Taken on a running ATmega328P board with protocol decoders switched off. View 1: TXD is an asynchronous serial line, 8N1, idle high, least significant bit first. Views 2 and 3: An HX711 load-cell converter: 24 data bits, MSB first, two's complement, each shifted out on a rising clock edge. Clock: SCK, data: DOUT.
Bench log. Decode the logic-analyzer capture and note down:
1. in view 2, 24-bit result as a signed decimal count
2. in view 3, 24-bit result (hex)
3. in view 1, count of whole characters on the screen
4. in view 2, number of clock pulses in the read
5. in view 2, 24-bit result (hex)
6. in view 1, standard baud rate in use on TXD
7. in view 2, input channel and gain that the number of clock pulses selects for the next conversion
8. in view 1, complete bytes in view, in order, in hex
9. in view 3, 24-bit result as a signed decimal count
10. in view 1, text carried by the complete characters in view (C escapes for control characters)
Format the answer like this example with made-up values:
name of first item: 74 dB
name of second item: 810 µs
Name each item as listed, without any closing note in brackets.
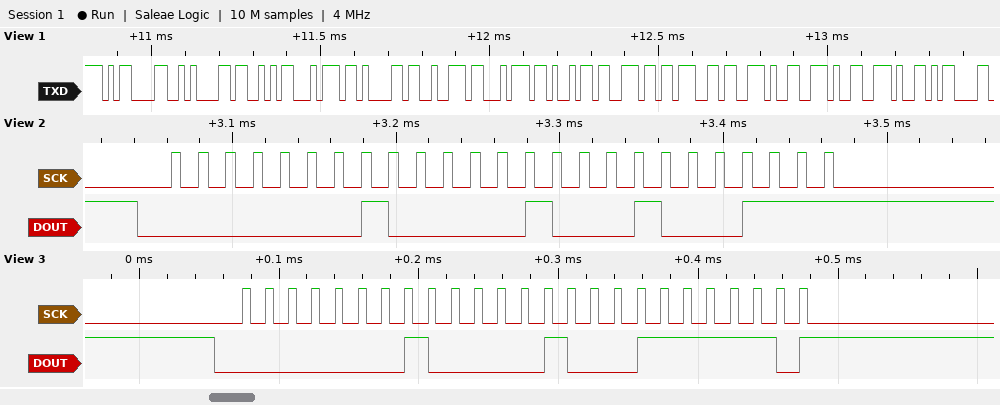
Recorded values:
in view 2, 24-bit result as a signed decimal count: 66631
in view 3, 24-bit result: 0x01047E
in view 1, count of whole characters on the screen: 14
in view 2, number of clock pulses in the read: 25
in view 2, 24-bit result: 0x010447
in view 1, standard baud rate in use on TXD: 57600 baud
in view 2, input channel and gain that the number of clock pulses selects for the next conversion: channel A, gain 128
in view 1, complete bytes in view, in order, in hex: 0x0D 0x0A 0x53 0x74 0x61 0x72 0x74 0x69 0x6E 0x67 0x2E 0x2E 0x2E 0x0D
in view 3, 24-bit result as a signed decimal count: 66686
in view 1, text carried by the complete characters in view: "\r\nStarting...\r"
